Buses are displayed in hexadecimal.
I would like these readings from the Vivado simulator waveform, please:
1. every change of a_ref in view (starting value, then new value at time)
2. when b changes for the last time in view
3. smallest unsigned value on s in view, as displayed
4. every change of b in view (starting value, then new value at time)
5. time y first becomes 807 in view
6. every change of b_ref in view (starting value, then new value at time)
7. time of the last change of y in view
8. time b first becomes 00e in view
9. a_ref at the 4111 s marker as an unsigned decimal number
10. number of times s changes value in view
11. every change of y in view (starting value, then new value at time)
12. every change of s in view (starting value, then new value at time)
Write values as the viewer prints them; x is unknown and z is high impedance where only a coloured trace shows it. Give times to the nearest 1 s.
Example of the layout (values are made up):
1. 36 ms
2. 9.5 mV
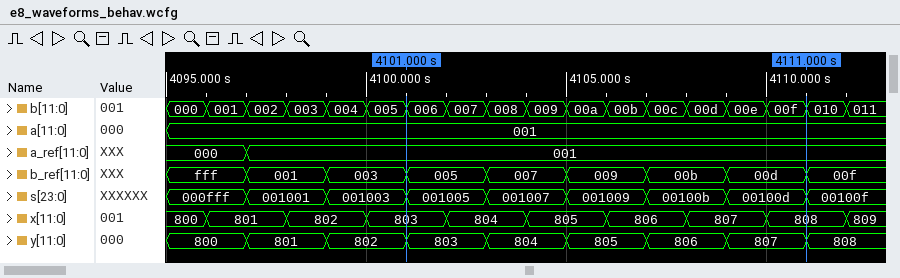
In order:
1. 000, 001 at 4097 s
2. 4112 s
3. 000fff
4. 000, 001 at 4096 s, 002 at 4097 s, 003 at 4098 s, 004 at 4099 s, 005 at 4100 s, 006 at 4101 s, 007 at 4102 s, 008 at 4103 s, 009 at 4104 s, 00a at 4105 s, 00b at 4106 s, 00c at 4107 s, 00d at 4108 s, 00e at 4109 s, 00f at 4110 s, 010 at 4111 s, 011 at 4112 s
5. 4109 s
6. fff, 001 at 4097 s, 003 at 4099 s, 005 at 4101 s, 007 at 4103 s, 009 at 4105 s, 00b at 4107 s, 00d at 4109 s, 00f at 4111 s
7. 4111 s
8. 4109 s
9. 1
10. 8
11. 800, 801 at 4097 s, 802 at 4099 s, 803 at 4101 s, 804 at 4103 s, 805 at 4105 s, 806 at 4107 s, 807 at 4109 s, 808 at 4111 s
12. 000fff, 001001 at 4097 s, 001003 at 4099 s, 001005 at 4101 s, 001007 at 4103 s, 001009 at 4105 s, 00100b at 4107 s, 00100d at 4109 s, 00100f at 4111 s
